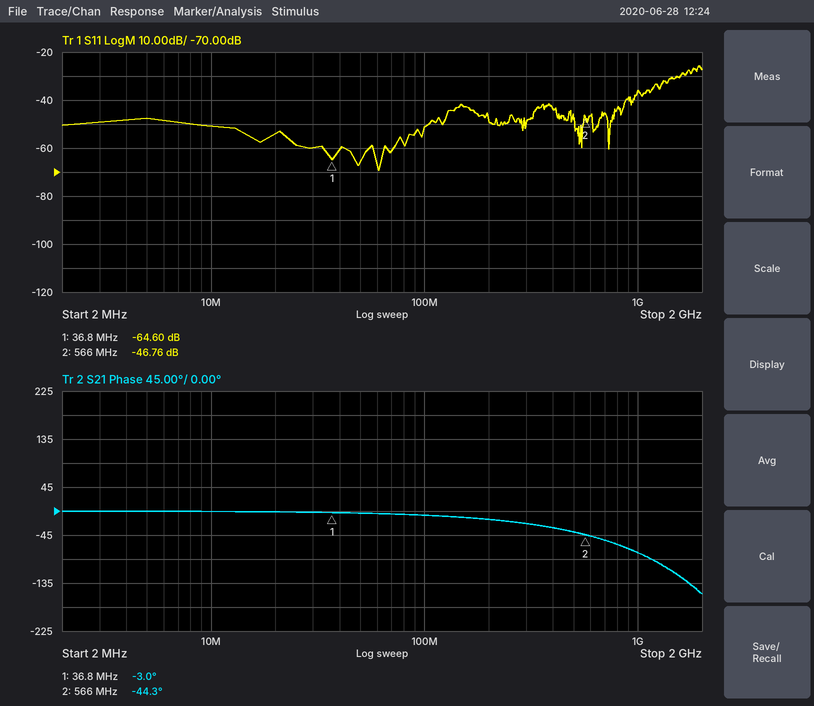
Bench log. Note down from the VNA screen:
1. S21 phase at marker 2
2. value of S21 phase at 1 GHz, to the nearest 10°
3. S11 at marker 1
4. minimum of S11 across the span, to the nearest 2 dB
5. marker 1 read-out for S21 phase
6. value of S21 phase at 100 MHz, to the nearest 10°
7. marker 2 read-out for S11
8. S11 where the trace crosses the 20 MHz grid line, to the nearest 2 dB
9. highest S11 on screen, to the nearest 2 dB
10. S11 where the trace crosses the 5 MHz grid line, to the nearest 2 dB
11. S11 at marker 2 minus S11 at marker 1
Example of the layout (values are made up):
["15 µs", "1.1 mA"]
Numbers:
["-44.3°", "-80°", "-64.60 dB", "-70 dB", "-3.0°", "-10°", "-46.76 dB", "-54 dB", "-26 dB", "-48 dB", "17.84 dB"]
